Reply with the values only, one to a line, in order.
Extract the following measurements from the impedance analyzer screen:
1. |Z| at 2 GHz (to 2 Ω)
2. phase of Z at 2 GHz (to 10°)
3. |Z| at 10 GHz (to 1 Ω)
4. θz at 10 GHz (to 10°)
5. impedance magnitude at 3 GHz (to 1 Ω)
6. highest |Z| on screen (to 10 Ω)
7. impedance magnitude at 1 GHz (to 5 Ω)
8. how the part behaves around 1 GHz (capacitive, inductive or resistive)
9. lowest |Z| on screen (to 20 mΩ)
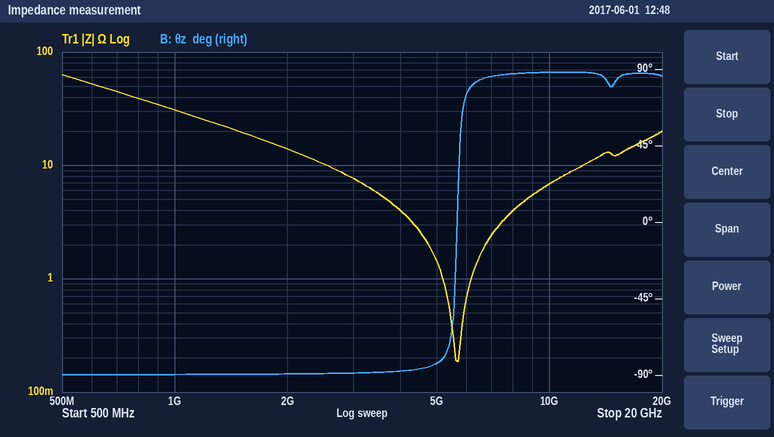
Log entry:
14 Ω
-90°
7 Ω
90°
8 Ω
60 Ω
30 Ω
capacitive
180 mΩ
